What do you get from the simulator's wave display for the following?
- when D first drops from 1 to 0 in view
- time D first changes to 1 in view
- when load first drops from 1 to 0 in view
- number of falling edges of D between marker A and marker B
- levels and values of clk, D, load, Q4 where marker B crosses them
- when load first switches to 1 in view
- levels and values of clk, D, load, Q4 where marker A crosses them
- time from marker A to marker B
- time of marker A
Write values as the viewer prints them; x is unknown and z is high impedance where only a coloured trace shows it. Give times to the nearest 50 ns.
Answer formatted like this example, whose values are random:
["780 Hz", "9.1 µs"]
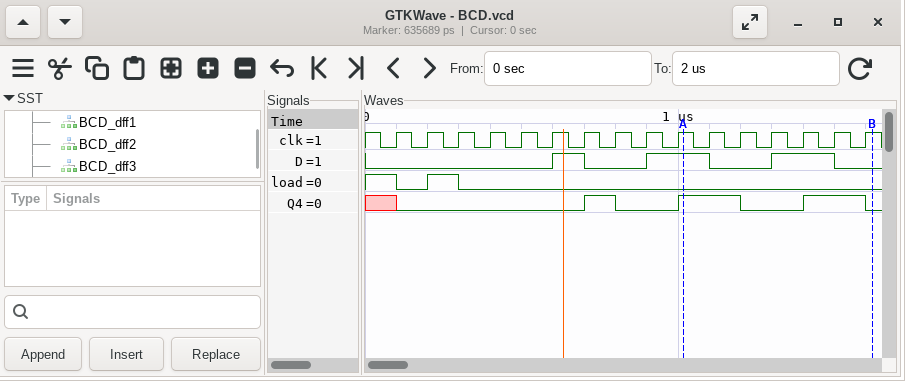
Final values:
["700 ns", "600 ns", "100 ns", "2", "clk=1, D=0, load=0, Q4=0", "200 ns", "clk=1, D=1, load=0, Q4=1", "600 ns", "1000 ns"]
